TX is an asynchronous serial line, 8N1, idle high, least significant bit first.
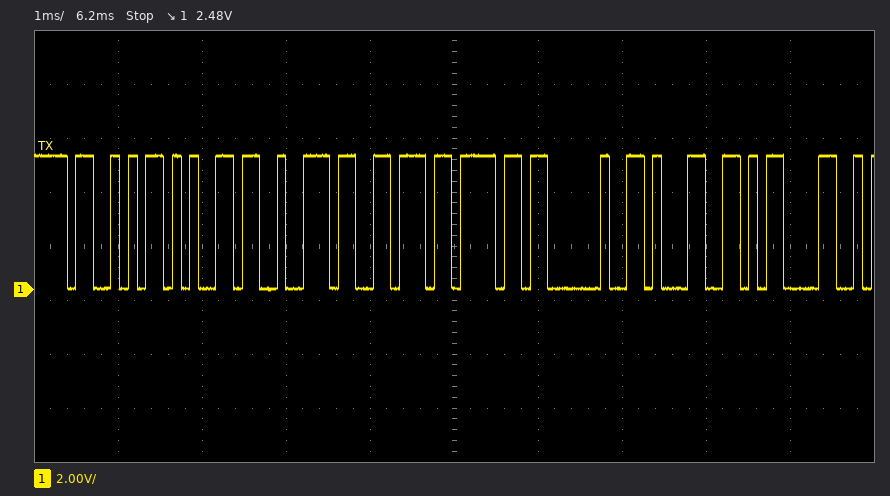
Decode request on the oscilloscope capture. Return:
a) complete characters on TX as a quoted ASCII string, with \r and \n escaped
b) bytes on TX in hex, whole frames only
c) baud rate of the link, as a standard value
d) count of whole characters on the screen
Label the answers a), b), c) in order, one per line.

a) "Servo 1\r"
b) 0x53 0x65 0x72 0x76 0x6F 0x20 0x31 0x0D
c) 9600 baud
d) 8
